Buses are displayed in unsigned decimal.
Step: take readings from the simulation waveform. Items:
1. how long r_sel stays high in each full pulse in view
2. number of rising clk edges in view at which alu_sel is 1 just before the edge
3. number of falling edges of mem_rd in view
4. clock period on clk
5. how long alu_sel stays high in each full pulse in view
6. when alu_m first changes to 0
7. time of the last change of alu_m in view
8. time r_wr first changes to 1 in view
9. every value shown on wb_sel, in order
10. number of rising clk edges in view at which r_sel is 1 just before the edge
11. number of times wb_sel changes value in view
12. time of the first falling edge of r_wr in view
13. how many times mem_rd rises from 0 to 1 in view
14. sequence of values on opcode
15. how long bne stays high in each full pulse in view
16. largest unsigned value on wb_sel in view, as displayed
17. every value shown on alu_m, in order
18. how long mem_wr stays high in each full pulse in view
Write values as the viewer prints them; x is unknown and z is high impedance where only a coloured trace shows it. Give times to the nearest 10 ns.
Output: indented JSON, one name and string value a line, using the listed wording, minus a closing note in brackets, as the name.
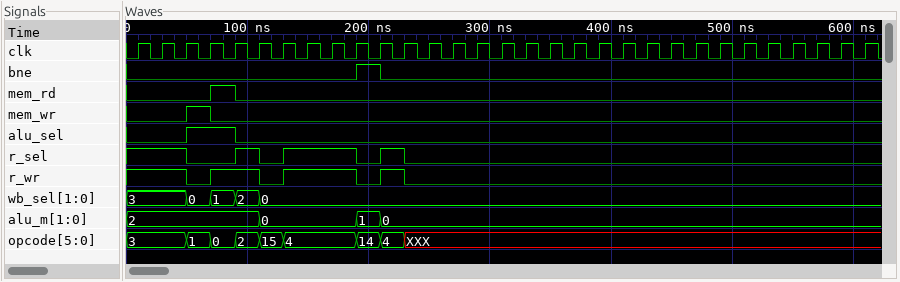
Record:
{
  "how long r_sel stays high in each full pulse in view": "20 ns, 60 ns, 20 ns",
  "number of rising clk edges in view at which alu_sel is 1 just before the edge": "2",
  "number of falling edges of mem_rd in view": "1",
  "clock period on clk": "20 ns",
  "how long alu_sel stays high in each full pulse in view": "40 ns",
  "when alu_m first changes to 0": "110 ns",
  "time of the last change of alu_m in view": "210 ns",
  "time r_wr first changes to 1 in view": "70 ns",
  "every value shown on wb_sel, in order": "3, 0, 1, 2, 0",
  "number of rising clk edges in view at which r_sel is 1 just before the edge": "8",
  "number of times wb_sel changes value in view": "4",
  "time of the first falling edge of r_wr in view": "50 ns",
  "how many times mem_rd rises from 0 to 1 in view": "1",
  "sequence of values on opcode": "3, 1, 0, 2, 15, 4, 14, 4, XXX",
  "how long bne stays high in each full pulse in view": "20 ns",
  "largest unsigned value on wb_sel in view, as displayed": "3",
  "every value shown on alu_m, in order": "2, 0, 1, 0",
  "how long mem_wr stays high in each full pulse in view": "20 ns"
}
